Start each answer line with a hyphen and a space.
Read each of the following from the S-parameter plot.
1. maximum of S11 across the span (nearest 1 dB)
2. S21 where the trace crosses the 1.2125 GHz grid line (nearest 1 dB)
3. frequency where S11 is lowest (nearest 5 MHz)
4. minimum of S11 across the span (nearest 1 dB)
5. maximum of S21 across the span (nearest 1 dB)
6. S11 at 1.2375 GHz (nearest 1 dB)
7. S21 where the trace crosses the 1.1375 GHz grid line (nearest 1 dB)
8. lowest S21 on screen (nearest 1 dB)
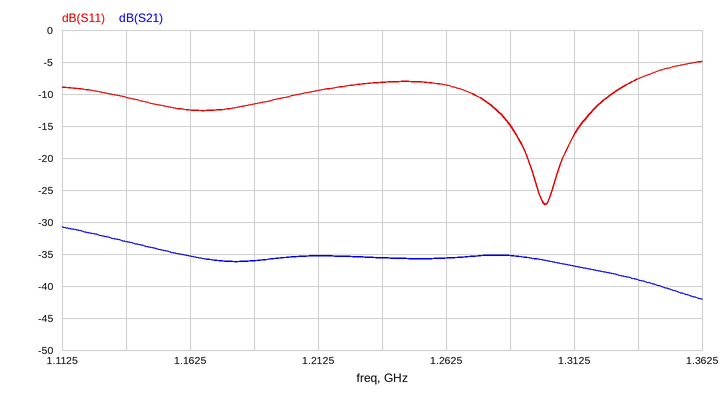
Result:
- -5 dB
- -35 dB
- 1.300 GHz
- -27 dB
- -31 dB
- -8 dB
- -33 dB
- -42 dB
